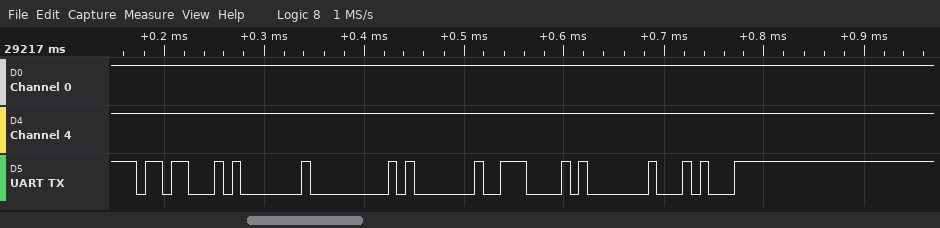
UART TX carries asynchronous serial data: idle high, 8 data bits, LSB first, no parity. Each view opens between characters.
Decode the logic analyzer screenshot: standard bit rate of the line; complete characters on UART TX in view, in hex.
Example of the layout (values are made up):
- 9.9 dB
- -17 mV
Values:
- 115200 baud
- 1B, 01, 00, 01, 0E, 01, 14
